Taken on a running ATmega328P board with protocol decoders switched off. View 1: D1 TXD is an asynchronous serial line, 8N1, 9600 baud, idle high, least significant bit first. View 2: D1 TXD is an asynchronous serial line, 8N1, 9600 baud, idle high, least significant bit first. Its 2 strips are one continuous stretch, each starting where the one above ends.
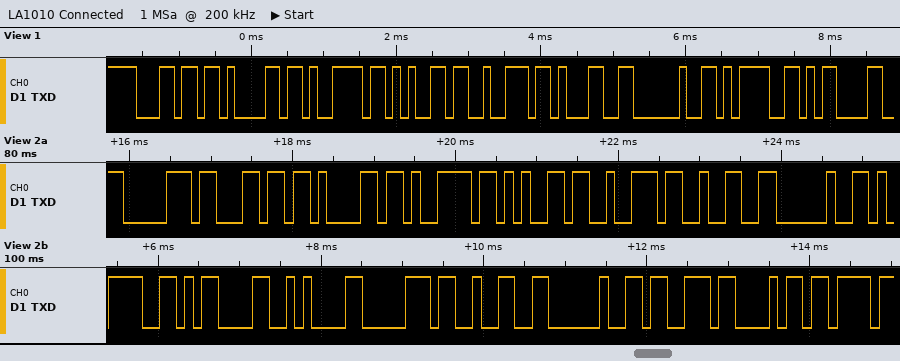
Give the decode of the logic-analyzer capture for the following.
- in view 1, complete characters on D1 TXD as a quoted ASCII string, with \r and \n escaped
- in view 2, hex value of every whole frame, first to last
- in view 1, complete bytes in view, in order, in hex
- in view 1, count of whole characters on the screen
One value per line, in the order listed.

"layer1 =\r"
70 6C 61 79 65 72 32 20 3D 0D 0A 70 32 20 73 68
6C 61 79 65 72 31 20 3D 0D
9
